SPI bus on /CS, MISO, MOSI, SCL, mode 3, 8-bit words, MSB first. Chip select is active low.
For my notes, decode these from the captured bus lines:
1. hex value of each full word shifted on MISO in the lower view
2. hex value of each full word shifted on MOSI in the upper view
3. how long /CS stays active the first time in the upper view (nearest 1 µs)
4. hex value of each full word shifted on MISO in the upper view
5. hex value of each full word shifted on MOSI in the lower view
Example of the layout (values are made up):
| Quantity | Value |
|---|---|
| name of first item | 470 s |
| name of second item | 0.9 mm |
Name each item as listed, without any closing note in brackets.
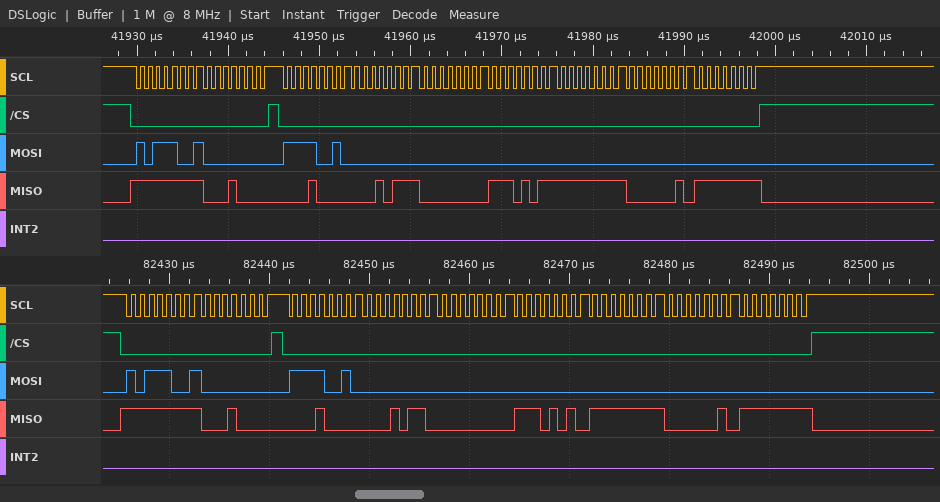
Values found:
| Quantity | Value |
|---|---|
| hex value of each full word shifted on MISO in the lower view | FF, 10, 10, 16, 00, EA, FF, 02, FF |
| hex value of each full word shifted on MOSI in the upper view | B9, 00, F2, 00, 00, 00, 00, 00, 00 |
| how long /CS stays active the first time in the upper view | 15 µs |
| hex value of each full word shifted on MISO in the upper view | FF, 10, 10, 17, 00, EB, FF, 02, FF |
| hex value of each full word shifted on MOSI in the lower view | B9, 00, F2, 00, 00, 00, 00, 00, 00 |
